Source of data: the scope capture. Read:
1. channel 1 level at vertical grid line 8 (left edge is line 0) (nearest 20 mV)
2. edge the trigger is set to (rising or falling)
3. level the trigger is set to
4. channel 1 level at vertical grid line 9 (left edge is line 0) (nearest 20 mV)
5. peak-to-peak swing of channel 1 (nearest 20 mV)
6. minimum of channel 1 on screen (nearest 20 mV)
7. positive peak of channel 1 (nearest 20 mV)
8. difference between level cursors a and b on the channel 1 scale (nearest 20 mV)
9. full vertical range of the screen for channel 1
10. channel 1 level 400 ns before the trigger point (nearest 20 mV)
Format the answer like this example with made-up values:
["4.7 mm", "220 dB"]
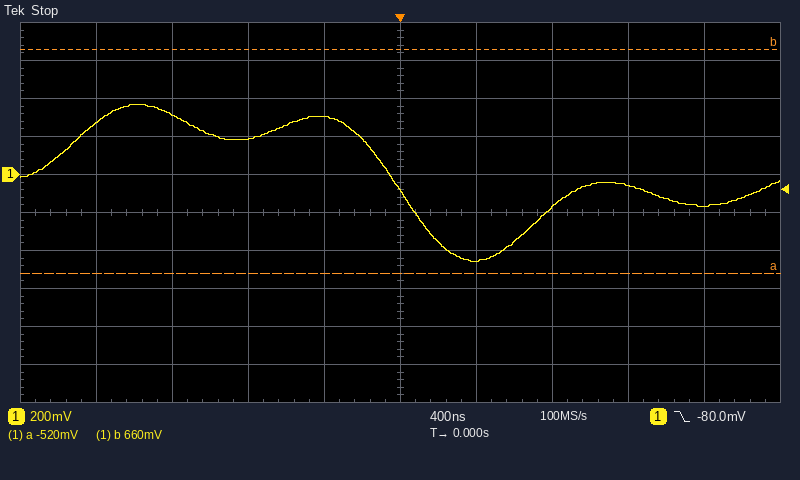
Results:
["-60 mV", "falling", "-80.0 mV", "-160 mV", "820 mV", "-460 mV", "360 mV", "1.18 V", "2 V", "300 mV"]
